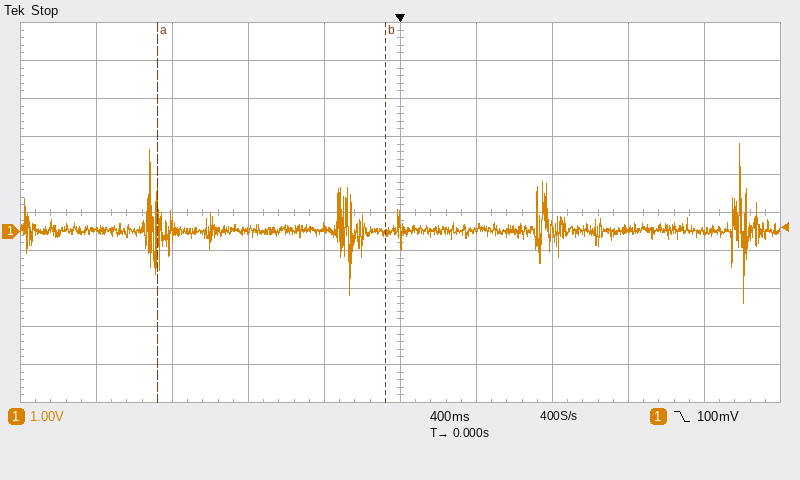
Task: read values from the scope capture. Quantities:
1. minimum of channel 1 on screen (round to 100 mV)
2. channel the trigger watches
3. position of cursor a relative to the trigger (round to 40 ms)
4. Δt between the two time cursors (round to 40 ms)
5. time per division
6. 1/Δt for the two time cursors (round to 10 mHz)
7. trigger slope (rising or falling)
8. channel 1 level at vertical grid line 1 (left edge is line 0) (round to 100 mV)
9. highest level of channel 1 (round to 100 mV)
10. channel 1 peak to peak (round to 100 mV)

-1.9 V
channel 1
-1.28 s
1.20 s
400 ms
830 mHz
falling
0.0 V
2.3 V
4.2 V
